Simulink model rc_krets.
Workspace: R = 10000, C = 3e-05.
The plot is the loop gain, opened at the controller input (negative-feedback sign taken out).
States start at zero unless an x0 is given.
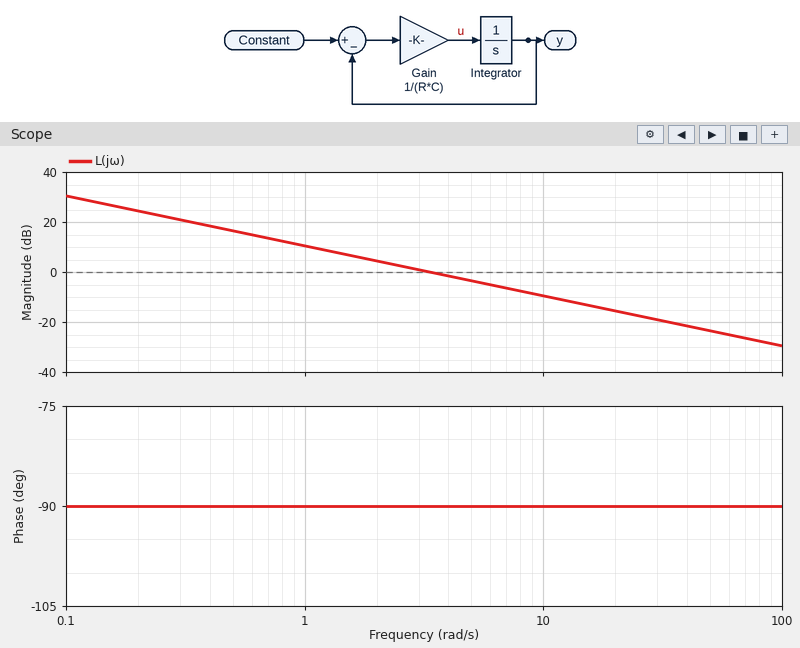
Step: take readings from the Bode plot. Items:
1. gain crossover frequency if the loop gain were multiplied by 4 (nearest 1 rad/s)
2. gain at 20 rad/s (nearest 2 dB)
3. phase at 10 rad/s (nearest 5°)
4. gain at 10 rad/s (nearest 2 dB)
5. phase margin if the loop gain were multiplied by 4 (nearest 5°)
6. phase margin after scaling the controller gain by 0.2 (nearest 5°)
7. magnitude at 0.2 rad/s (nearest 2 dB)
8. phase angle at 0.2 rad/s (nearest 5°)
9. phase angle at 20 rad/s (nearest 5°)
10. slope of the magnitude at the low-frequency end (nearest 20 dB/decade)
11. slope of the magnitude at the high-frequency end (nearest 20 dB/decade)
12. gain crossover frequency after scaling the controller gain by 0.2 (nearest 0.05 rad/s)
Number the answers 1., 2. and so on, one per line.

1. 13 rad/s
2. -16 dB
3. -90°
4. -10 dB
5. 90°
6. 90°
7. 24 dB
8. -90°
9. -90°
10. -20 dB/decade
11. -20 dB/decade
12. 0.65 rad/s
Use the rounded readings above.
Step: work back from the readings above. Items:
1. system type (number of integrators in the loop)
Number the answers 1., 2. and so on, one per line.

1. 1
